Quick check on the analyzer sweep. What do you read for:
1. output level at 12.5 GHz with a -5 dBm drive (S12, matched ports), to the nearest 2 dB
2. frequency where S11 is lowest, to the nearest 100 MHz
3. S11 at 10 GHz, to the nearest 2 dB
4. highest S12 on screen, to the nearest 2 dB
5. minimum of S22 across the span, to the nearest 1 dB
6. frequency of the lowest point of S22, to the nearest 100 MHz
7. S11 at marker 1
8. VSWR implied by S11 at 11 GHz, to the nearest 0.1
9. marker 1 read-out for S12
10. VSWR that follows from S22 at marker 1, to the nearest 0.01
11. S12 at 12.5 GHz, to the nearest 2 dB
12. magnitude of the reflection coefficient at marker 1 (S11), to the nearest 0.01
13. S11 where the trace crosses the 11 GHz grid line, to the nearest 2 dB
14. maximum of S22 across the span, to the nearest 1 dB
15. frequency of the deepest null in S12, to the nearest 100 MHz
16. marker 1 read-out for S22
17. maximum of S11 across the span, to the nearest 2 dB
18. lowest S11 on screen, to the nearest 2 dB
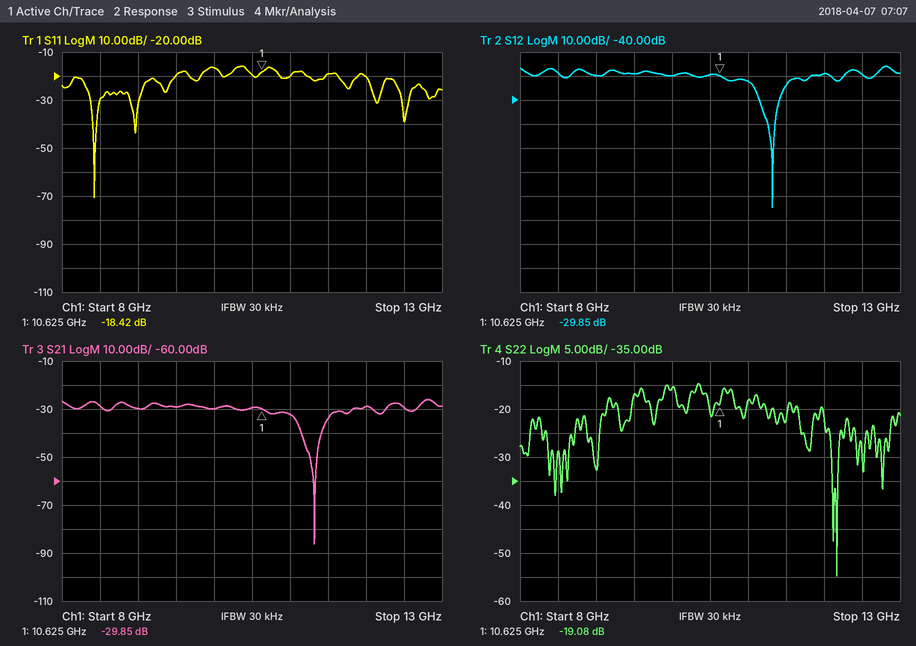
-34 dBm
8.4 GHz
-16 dB
-26 dB
-55 dB
12.2 GHz
-18.42 dB
1.2
-29.85 dB
1.25
-30 dB
0.12
-20 dB
-15 dB
11.3 GHz
-19.08 dB
-16 dB
-70 dB
